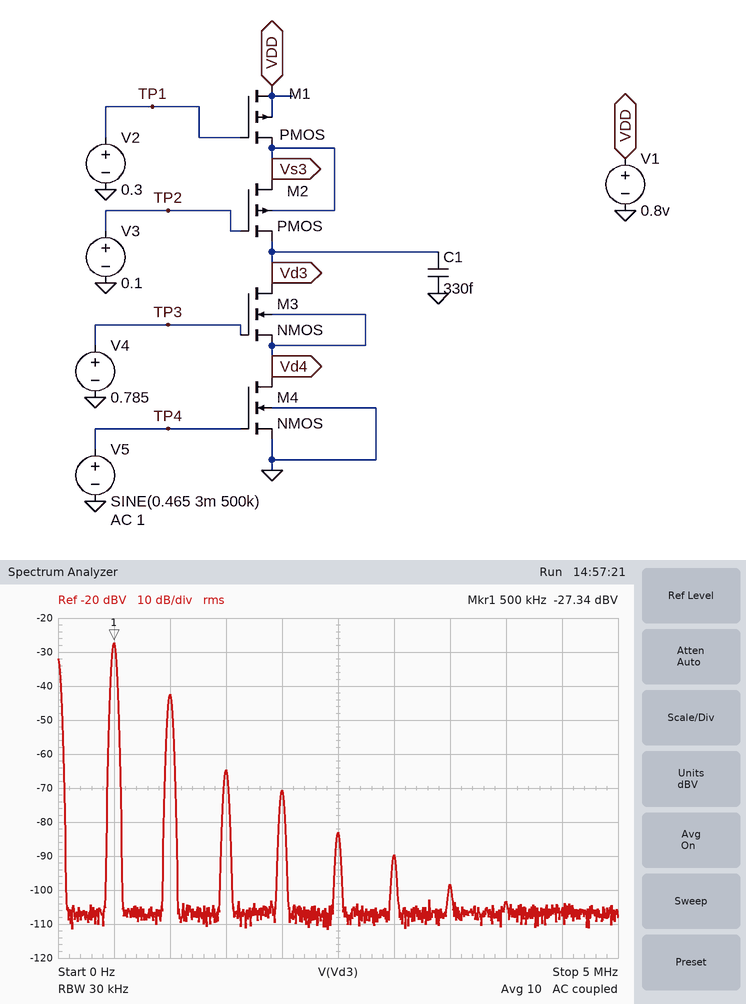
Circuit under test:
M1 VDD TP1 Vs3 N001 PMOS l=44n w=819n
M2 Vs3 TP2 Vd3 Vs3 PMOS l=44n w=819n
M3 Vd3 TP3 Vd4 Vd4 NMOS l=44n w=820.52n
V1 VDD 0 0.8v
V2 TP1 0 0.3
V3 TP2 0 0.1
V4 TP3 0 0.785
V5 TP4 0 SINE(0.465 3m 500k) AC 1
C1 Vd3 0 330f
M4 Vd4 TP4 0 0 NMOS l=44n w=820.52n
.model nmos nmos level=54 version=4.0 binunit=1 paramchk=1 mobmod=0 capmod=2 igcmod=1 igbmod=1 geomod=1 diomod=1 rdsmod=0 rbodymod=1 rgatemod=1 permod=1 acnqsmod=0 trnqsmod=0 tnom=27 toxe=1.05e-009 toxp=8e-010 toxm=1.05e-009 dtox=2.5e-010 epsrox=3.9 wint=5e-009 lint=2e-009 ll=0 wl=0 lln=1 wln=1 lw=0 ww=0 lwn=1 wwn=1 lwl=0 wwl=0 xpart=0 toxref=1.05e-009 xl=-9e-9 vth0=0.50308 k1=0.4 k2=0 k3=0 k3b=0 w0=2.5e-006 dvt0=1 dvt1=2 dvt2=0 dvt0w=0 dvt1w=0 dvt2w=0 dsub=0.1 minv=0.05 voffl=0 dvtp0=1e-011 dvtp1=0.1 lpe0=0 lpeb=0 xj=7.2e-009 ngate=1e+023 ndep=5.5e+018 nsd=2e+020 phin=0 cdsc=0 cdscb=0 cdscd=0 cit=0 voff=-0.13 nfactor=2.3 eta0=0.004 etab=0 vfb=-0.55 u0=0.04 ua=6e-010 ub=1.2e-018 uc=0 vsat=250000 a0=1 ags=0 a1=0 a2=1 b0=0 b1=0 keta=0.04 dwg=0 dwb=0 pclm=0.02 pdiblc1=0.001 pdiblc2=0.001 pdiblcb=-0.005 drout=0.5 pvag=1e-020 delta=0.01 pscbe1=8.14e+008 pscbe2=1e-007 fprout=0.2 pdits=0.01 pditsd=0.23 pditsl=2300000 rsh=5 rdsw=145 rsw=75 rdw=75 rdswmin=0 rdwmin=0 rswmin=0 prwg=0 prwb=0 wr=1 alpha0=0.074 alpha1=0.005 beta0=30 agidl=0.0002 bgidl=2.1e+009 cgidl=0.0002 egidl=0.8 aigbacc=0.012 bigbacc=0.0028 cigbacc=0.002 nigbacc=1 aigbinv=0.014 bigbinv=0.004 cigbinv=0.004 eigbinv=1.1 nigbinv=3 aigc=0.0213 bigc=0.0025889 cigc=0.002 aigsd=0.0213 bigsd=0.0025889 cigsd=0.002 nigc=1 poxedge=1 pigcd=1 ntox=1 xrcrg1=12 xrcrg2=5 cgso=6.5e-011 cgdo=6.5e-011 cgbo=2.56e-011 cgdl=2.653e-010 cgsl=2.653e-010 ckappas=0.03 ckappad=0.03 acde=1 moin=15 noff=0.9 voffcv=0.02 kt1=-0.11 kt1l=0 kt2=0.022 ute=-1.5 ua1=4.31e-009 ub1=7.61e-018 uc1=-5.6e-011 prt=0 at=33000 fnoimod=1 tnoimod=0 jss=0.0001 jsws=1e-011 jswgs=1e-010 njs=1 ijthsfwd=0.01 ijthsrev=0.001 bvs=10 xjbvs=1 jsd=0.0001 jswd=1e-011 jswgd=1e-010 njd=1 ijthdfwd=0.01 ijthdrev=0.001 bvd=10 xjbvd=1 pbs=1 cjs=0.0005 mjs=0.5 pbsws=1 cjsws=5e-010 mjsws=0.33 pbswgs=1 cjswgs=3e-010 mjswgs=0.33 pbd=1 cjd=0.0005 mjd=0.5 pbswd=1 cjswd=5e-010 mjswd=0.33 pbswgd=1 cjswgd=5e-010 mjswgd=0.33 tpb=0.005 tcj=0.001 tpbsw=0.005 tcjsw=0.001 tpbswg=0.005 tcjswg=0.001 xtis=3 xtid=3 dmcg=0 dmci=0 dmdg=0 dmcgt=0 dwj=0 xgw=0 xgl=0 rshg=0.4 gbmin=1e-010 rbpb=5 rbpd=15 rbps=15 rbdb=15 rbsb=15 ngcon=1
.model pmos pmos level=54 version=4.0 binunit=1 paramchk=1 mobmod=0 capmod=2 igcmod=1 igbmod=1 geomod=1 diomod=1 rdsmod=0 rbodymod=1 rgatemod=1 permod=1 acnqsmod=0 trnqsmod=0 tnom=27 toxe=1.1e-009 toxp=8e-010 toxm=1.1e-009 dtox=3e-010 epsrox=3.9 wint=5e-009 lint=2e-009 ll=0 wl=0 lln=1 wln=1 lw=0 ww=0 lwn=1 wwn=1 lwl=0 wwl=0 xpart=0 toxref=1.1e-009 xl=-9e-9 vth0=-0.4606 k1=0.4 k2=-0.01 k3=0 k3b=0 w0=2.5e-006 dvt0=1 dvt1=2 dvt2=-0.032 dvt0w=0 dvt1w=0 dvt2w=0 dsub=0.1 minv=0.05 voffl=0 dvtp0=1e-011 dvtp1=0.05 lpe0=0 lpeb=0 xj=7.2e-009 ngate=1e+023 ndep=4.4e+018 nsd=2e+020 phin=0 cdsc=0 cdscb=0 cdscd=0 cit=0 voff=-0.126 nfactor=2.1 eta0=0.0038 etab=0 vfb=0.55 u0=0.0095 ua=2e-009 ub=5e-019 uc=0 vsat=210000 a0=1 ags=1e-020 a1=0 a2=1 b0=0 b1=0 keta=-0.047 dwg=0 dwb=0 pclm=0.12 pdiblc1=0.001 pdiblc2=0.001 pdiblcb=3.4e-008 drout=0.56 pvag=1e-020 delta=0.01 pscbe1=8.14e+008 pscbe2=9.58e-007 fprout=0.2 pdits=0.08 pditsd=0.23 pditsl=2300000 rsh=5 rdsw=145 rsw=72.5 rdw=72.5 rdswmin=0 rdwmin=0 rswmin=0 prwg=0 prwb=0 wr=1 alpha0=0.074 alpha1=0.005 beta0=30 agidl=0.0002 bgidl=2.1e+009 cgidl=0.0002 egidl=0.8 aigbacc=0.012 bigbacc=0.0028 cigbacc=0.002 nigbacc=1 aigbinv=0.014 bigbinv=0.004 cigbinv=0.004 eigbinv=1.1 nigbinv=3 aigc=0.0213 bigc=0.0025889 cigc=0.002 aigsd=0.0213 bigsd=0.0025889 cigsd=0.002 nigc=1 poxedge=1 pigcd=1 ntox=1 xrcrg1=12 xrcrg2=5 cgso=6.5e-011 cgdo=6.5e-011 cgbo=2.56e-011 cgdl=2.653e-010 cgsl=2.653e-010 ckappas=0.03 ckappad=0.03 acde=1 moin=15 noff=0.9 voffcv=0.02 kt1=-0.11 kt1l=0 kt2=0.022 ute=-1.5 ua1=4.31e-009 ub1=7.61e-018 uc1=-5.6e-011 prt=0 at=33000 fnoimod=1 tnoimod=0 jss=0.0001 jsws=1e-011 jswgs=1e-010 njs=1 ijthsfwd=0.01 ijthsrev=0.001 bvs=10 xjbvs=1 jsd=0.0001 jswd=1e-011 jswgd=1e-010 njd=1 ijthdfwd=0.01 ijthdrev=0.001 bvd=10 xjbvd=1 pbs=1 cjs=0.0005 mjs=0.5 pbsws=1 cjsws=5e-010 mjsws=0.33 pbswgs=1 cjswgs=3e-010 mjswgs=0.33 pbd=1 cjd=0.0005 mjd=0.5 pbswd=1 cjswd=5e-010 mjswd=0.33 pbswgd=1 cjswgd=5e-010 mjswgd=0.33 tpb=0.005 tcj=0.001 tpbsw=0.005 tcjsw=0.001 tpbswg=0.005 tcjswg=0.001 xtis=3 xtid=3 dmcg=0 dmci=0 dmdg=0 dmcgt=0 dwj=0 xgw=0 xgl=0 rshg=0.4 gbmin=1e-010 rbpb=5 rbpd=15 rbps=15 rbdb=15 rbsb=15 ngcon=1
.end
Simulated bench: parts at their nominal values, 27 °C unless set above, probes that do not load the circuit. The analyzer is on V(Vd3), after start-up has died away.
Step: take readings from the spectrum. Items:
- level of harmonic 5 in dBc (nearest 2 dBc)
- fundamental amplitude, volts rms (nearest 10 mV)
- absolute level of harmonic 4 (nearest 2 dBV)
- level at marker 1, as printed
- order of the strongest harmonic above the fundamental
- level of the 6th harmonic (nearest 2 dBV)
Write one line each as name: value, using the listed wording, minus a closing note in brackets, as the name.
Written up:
level of harmonic 5 in dBc: -56 dBc
fundamental amplitude, volts rms: 40 mV
absolute level of harmonic 4: -70 dBV
level at marker 1, as printed: -27.34 dBV
order of the strongest harmonic above the fundamental: 2
level of the 6th harmonic: -90 dBV
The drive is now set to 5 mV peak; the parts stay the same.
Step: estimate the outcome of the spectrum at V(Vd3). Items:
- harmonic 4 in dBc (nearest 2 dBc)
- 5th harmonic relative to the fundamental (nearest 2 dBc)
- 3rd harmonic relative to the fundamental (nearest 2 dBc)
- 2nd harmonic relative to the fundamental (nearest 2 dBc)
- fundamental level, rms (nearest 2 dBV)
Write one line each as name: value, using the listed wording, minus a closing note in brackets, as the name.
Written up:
harmonic 4 in dBc: -36 dBc
5th harmonic relative to the fundamental: -48 dBc
3rd harmonic relative to the fundamental: -32 dBc
2nd harmonic relative to the fundamental: -12 dBc
fundamental level, rms: -22 dBV
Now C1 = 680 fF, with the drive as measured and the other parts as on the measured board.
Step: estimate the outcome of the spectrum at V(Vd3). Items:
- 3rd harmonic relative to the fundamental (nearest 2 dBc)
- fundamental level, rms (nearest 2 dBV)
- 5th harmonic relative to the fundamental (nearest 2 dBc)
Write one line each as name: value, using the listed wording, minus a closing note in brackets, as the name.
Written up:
3rd harmonic relative to the fundamental: -34 dBc
fundamental level, rms: -28 dBV
5th harmonic relative to the fundamental: -54 dBc
